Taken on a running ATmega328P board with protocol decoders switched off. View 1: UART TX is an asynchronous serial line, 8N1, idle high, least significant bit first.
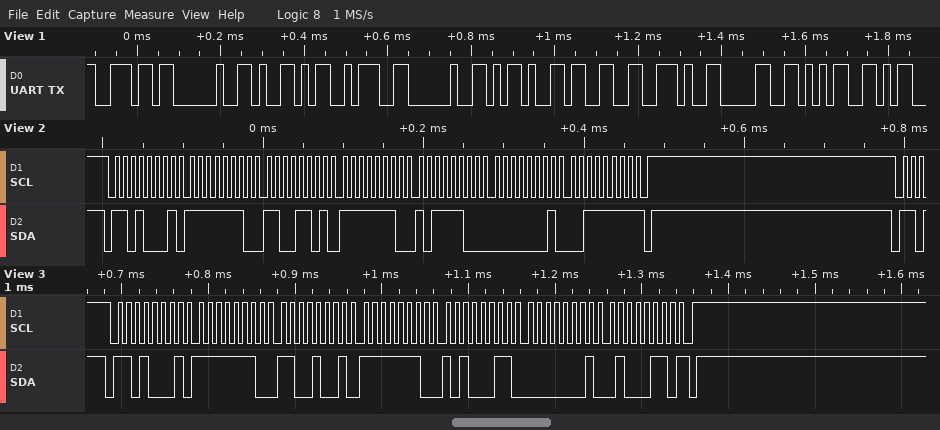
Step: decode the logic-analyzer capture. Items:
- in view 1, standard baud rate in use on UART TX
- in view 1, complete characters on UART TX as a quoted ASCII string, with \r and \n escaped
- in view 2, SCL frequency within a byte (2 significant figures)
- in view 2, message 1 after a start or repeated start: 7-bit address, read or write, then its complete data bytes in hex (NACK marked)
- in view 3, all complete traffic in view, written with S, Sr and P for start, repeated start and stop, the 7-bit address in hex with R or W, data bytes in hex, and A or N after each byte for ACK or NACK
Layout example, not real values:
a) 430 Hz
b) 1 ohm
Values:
a) 57600 baud
b) "n Y: -3.05"
c) 100 kHz
d) 0x68 read: FE CD FE BC 01 3F NACK
e) S 68R A FE A C9 A FE A A3 A 01 A 46 N P
